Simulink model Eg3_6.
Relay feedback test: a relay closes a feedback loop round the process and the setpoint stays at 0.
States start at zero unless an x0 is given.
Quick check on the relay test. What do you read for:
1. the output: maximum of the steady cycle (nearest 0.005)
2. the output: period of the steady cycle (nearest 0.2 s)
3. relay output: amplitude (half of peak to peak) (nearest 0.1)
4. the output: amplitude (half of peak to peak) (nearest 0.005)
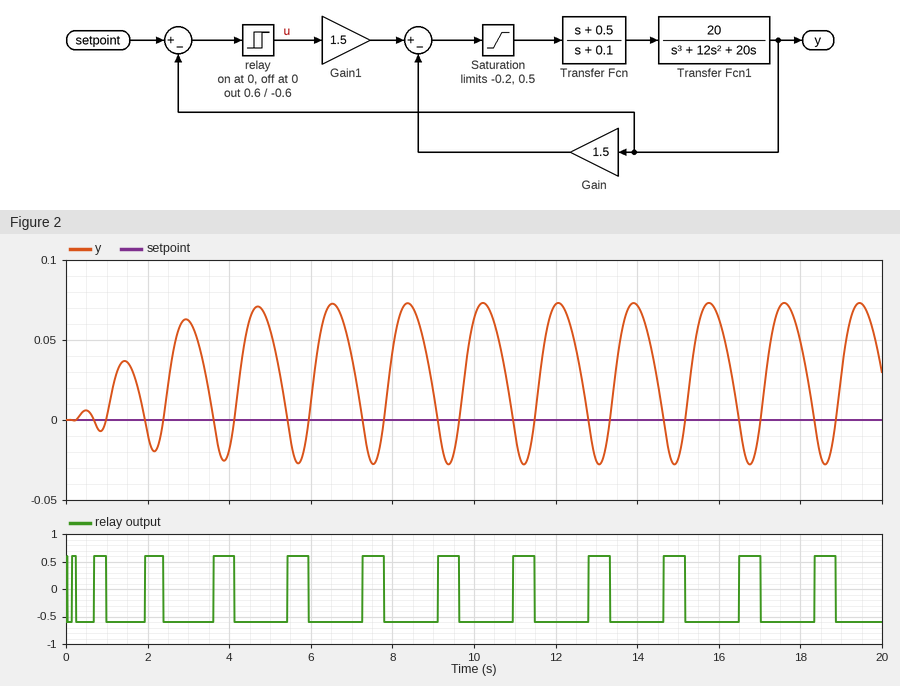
0.075
1.8 s
0.6
0.050
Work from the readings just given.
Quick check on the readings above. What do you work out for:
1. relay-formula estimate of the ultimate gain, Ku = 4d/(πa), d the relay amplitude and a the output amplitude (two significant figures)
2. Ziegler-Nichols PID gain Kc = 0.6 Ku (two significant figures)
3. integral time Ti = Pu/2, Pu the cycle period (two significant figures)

15
9.0
0.90 s
